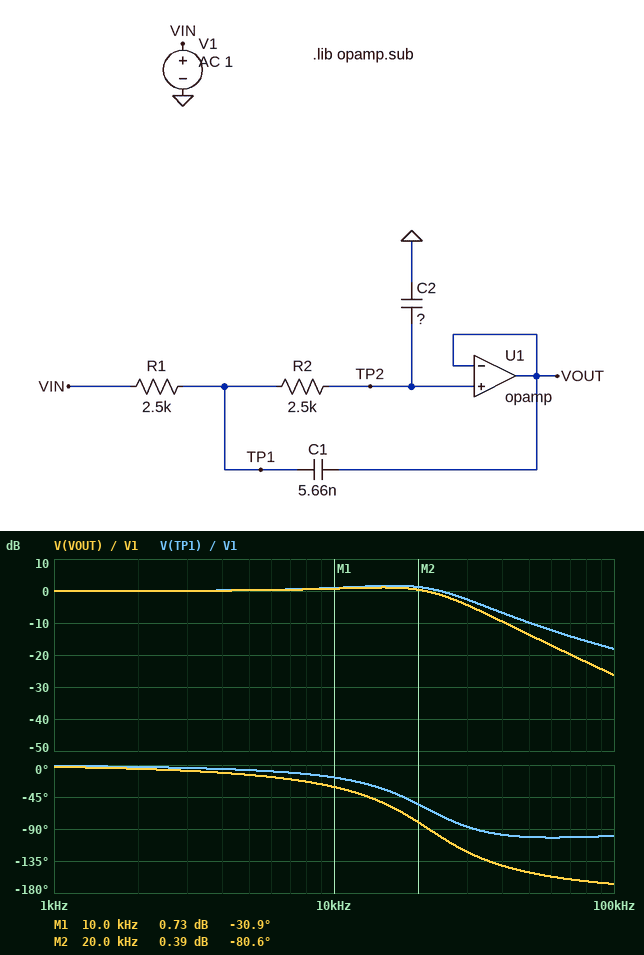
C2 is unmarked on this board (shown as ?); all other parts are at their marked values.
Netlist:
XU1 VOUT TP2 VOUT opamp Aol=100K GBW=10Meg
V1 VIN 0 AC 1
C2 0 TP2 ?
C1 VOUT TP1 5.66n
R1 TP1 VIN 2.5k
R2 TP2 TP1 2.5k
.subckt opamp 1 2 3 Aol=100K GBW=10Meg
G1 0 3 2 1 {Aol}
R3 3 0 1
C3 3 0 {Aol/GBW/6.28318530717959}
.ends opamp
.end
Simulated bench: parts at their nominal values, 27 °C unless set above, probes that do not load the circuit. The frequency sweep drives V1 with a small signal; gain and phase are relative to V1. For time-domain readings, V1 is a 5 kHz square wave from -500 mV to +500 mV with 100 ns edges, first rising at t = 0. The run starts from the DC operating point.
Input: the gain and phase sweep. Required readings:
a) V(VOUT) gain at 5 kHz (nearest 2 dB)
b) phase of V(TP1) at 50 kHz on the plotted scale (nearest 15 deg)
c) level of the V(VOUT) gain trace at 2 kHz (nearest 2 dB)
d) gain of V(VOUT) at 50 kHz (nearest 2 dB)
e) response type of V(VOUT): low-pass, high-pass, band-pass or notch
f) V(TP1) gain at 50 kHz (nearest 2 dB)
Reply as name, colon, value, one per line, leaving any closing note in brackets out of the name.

V(VOUT) gain at 5 kHz: 0 dB
phase of V(TP1) at 50 kHz on the plotted scale: -105 deg
level of the V(VOUT) gain trace at 2 kHz: 0 dB
gain of V(VOUT) at 50 kHz: -14 dB
response type of V(VOUT): low-pass, high-pass, band-pass or notch: low-pass
V(TP1) gain at 50 kHz: -10 dB
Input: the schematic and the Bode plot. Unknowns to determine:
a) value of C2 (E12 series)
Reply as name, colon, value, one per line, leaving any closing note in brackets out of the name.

value of C2: 1.5 nF
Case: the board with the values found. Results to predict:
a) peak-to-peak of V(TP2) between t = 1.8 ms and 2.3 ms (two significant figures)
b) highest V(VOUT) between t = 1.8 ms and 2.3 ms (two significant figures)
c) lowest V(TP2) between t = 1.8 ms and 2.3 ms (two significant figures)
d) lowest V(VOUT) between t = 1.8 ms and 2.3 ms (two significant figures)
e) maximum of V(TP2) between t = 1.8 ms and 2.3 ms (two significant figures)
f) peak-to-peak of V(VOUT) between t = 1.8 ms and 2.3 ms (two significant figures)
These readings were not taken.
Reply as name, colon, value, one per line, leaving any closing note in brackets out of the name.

peak-to-peak of V(TP2) between t = 1.8 ms and 2.3 ms: 1.3 V
highest V(VOUT) between t = 1.8 ms and 2.3 ms: 650 mV
lowest V(TP2) between t = 1.8 ms and 2.3 ms: -650 mV
lowest V(VOUT) between t = 1.8 ms and 2.3 ms: -650 mV
maximum of V(TP2) between t = 1.8 ms and 2.3 ms: 650 mV
peak-to-peak of V(VOUT) between t = 1.8 ms and 2.3 ms: 1.3 V
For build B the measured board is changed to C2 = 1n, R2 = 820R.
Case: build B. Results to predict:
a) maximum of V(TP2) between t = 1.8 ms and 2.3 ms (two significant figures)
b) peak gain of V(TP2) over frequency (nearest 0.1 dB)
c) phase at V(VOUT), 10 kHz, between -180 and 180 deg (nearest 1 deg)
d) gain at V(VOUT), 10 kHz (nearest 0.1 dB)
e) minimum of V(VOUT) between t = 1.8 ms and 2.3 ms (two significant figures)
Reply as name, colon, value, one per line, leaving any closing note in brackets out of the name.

maximum of V(TP2) between t = 1.8 ms and 2.3 ms: 680 mV
peak gain of V(TP2) over frequency: 1.5 dB
phase at V(VOUT), 10 kHz, between -180 and 180 deg: -12 deg
gain at V(VOUT), 10 kHz: 0.2 dB
minimum of V(VOUT) between t = 1.8 ms and 2.3 ms: -680 mV
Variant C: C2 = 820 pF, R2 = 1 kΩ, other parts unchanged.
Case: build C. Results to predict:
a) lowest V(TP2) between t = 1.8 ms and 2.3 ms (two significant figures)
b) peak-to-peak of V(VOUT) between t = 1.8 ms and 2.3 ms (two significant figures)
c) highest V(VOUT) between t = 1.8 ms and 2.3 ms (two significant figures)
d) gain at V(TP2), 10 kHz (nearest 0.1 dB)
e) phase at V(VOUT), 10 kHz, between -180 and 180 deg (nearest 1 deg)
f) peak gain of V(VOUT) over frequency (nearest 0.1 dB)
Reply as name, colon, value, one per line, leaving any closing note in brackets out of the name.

lowest V(TP2) between t = 1.8 ms and 2.3 ms: -740 mV
peak-to-peak of V(VOUT) between t = 1.8 ms and 2.3 ms: 1.5 V
highest V(VOUT) between t = 1.8 ms and 2.3 ms: 740 mV
gain at V(TP2), 10 kHz: 0.3 dB
phase at V(VOUT), 10 kHz, between -180 and 180 deg: -11 deg
peak gain of V(VOUT) over frequency: 2.4 dB
